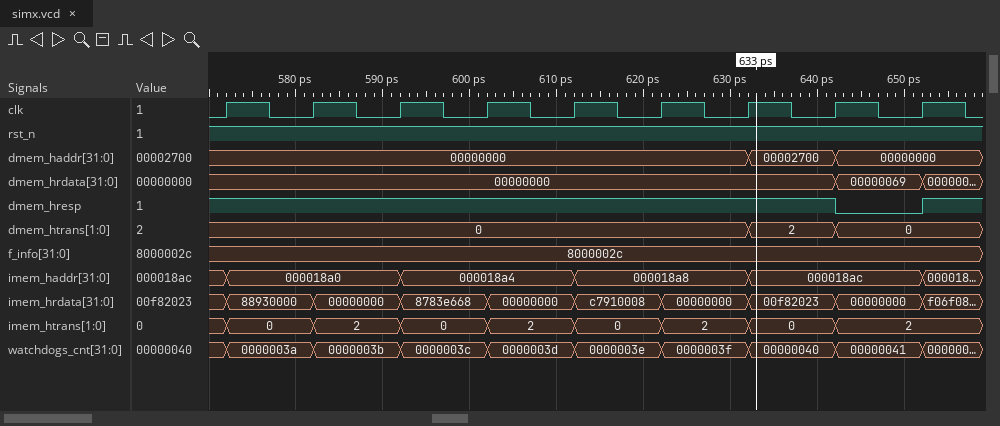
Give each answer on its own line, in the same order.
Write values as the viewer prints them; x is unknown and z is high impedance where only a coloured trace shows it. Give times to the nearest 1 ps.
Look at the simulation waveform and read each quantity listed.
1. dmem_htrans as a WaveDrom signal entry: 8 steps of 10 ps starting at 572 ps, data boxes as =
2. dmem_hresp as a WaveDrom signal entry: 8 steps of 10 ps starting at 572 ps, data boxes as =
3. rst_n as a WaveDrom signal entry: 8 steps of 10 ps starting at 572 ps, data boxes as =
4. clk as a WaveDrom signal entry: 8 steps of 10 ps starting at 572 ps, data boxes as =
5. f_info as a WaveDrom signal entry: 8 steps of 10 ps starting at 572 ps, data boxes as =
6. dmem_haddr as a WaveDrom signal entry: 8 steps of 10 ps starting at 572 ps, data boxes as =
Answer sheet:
{name: 'dmem_htrans', wave: '=.....==', data: '0 2 0'}
{name: 'dmem_hresp', wave: '1......0'}
{name: 'rst_n', wave: '1.......'}
{name: 'clk', wave: 'p.......'}
{name: 'f_info', wave: '=.......', data: '8000002c'}
{name: 'dmem_haddr', wave: '=.....==', data: '00000000 00002700 00000000'}
